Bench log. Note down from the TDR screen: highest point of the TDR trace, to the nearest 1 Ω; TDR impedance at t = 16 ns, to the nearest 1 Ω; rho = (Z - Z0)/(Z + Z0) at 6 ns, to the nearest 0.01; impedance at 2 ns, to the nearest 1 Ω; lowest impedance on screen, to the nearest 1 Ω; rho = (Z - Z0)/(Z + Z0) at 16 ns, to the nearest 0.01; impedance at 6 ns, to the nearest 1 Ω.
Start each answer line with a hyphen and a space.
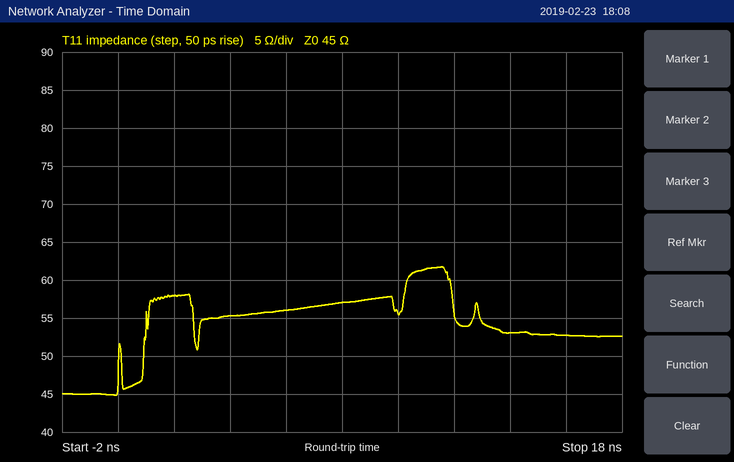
- 62 Ω
- 53 Ω
- +0.11
- 58 Ω
- 45 Ω
- +0.08
- 56 Ω
